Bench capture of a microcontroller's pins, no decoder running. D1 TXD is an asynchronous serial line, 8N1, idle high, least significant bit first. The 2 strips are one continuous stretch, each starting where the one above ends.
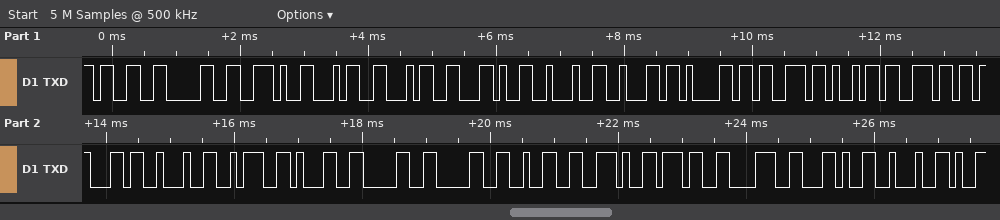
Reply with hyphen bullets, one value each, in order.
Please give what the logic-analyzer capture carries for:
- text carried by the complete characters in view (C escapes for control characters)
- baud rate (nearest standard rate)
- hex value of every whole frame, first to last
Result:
- "30.44,\"basinc\":1002.78,\""
- 9600 baud
- 33 30 2E 34 34 2C 22 62 61 73 69 6E 63 22 3A 31 30 30 32 2E 37 38 2C 22
